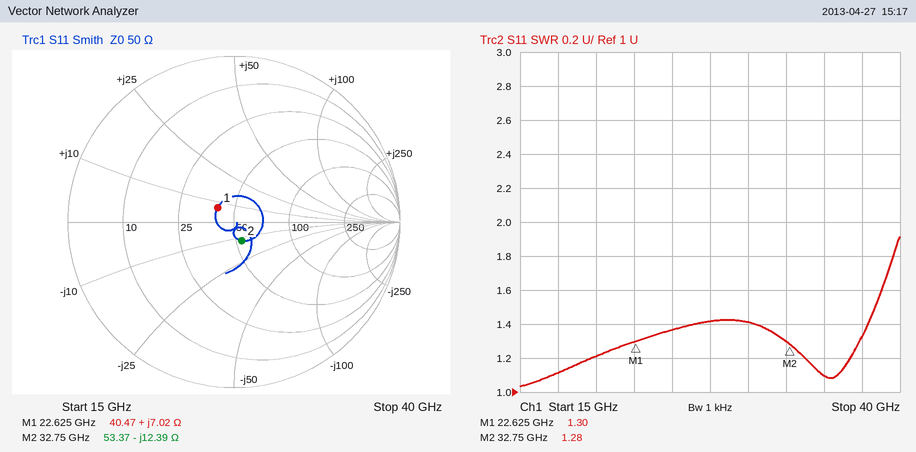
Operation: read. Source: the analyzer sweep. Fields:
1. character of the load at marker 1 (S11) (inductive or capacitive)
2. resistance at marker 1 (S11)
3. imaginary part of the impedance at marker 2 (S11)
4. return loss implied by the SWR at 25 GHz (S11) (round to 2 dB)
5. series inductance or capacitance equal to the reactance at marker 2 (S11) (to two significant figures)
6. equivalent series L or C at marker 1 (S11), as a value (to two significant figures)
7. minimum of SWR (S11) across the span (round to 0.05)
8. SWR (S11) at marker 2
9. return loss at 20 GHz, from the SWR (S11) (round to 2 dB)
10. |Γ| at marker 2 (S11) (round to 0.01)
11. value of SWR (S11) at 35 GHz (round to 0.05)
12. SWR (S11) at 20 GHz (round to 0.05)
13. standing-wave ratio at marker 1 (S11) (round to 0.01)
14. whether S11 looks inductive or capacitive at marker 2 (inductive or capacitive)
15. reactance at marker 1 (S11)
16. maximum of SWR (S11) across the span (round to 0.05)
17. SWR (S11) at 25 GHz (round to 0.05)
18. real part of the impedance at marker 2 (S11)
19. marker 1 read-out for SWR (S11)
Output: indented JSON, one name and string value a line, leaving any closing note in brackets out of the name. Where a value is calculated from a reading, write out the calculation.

{
  "character of the load at marker 1 (S11)": "inductive",
  "resistance at marker 1": "40.47 Ω",
  "imaginary part of the impedance at marker 2": "-12.39 Ω",
  "return loss implied by the SWR at 25 GHz (S11)": "−20 log10((1.35 − 1)/(1.35 + 1)) ≈ 16 dB",
  "series inductance or capacitance equal to the reactance at marker 2 (S11)": "C = 1/(2π × 32.75 GHz × 12.39 Ω) ≈ 392 fF, so 390 fF to two significant figures",
  "equivalent series L or C at marker 1 (S11), as a value": "L = 7.02 Ω/(2π × 22.625 GHz) ≈ 49 pH",
  "minimum of SWR (S11) across the span": "1.05",
  "SWR (S11) at marker 2": "1.28",
  "return loss at 20 GHz, from the SWR (S11)": "−20 log10((1.2 − 1)/(1.2 + 1)) ≈ 20.8 dB, so 20 dB to the nearest 2 dB",
  "|Γ| at marker 2 (S11)": "0.12",
  "value of SWR (S11) at 35 GHz": "1.10",
  "SWR (S11) at 20 GHz": "1.20",
  "standing-wave ratio at marker 1 (S11)": "1.30",
  "whether S11 looks inductive or capacitive at marker 2": "capacitive",
  "reactance at marker 1": "+7.02 Ω",
  "maximum of SWR (S11) across the span": "1.90",
  "SWR (S11) at 25 GHz": "1.35",
  "real part of the impedance at marker 2": "53.37 Ω",
  "marker 1 read-out for SWR": "1.30"
}
